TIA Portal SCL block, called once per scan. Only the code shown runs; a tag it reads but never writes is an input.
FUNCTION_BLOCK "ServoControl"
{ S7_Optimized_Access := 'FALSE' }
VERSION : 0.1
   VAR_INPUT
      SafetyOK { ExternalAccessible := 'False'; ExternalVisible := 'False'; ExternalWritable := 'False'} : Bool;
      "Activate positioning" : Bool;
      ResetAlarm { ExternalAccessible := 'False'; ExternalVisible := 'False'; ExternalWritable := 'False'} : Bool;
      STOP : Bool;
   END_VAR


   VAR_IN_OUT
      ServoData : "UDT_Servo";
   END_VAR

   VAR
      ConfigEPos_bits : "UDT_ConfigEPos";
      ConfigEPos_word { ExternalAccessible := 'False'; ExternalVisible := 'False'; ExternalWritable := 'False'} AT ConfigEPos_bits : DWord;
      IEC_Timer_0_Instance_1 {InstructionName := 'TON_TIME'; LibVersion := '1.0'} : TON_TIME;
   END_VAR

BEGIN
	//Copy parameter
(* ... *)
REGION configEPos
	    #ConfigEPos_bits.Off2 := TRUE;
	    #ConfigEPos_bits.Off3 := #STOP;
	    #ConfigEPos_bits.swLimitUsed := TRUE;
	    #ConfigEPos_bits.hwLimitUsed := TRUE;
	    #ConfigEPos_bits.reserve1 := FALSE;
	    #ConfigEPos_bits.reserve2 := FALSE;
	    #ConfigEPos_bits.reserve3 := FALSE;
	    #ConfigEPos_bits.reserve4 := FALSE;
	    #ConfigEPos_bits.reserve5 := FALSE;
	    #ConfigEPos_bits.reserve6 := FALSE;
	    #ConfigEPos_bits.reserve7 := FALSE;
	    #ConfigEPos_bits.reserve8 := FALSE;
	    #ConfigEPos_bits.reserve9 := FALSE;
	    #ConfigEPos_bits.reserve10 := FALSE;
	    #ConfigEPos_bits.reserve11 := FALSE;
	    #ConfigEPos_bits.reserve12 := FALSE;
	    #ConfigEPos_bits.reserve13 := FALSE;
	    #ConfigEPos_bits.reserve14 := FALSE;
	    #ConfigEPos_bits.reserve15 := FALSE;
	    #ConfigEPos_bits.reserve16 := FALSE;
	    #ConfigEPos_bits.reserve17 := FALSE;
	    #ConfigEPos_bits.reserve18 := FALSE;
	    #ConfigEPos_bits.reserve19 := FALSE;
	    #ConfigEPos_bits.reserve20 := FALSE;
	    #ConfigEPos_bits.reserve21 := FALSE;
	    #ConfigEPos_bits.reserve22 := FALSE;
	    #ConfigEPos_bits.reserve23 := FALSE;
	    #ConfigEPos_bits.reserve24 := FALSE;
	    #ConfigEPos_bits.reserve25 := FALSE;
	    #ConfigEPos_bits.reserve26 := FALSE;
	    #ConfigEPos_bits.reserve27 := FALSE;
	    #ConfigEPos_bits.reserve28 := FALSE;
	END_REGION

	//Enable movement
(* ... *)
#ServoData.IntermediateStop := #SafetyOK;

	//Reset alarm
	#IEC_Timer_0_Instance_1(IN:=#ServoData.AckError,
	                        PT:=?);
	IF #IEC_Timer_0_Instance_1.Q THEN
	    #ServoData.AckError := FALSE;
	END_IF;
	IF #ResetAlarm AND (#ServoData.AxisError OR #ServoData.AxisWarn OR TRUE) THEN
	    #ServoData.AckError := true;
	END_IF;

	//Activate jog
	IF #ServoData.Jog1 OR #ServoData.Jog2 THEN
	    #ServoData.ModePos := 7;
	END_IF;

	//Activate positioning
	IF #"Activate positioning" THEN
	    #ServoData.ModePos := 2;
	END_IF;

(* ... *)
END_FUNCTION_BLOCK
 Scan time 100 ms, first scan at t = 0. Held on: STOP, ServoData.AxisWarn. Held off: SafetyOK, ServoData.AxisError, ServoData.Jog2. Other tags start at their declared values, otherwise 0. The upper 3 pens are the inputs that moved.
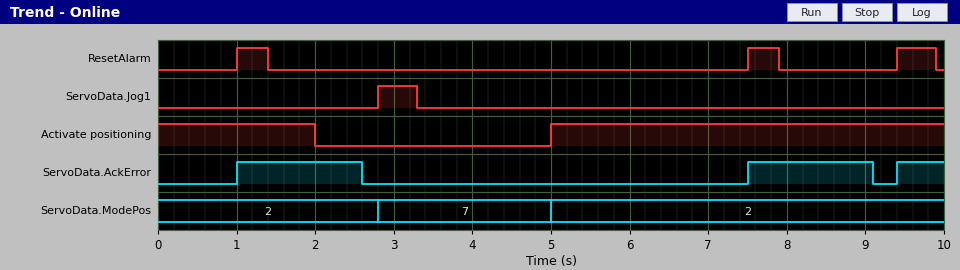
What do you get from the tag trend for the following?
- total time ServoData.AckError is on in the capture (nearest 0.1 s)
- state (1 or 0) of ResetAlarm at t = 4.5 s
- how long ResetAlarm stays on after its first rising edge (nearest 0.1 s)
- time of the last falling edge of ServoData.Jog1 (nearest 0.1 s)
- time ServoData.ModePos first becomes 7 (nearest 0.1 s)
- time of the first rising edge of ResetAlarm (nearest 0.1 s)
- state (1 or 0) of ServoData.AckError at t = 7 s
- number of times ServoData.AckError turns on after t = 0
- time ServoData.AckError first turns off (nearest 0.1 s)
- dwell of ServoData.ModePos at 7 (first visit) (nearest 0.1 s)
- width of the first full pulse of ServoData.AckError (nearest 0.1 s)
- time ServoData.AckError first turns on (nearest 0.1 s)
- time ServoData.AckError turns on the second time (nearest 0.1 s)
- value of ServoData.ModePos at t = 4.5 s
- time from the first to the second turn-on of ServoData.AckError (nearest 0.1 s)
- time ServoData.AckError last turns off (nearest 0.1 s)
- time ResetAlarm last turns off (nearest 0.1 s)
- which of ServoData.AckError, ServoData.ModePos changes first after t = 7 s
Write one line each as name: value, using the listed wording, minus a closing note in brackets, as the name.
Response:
total time ServoData.AckError is on in the capture: 3.8 s
state (1 or 0) of ResetAlarm at t = 4.5 s: 0
how long ResetAlarm stays on after its first rising edge: 0.4 s
time of the last falling edge of ServoData.Jog1: 3.3 s
time ServoData.ModePos first becomes 7: 2.8 s
time of the first rising edge of ResetAlarm: 1.0 s
state (1 or 0) of ServoData.AckError at t = 7 s: 0
number of times ServoData.AckError turns on after t = 0: 3
time ServoData.AckError first turns off: 2.6 s
dwell of ServoData.ModePos at 7 (first visit): 2.2 s
width of the first full pulse of ServoData.AckError: 1.6 s
time ServoData.AckError first turns on: 1.0 s
time ServoData.AckError turns on the second time: 7.5 s
value of ServoData.ModePos at t = 4.5 s: 7
time from the first to the second turn-on of ServoData.AckError: 6.5 s
time ServoData.AckError last turns off: 9.1 s
time ResetAlarm last turns off: 9.9 s
which of ServoData.AckError, ServoData.ModePos changes first after t = 7 s: ServoData.AckError
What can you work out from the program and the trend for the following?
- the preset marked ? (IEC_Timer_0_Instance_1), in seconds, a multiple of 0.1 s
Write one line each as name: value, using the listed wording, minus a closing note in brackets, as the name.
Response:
the preset marked ? (IEC_Timer_0_Instance_1), in seconds, a multiple of 0.1 s: 1.5 s
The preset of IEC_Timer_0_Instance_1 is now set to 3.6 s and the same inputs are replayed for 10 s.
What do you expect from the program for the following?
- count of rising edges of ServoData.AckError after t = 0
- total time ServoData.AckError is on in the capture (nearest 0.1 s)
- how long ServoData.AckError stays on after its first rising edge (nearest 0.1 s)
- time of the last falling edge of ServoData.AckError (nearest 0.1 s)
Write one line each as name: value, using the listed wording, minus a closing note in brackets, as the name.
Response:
count of rising edges of ServoData.AckError after t = 0: 2
total time ServoData.AckError is on in the capture: 6.2 s
how long ServoData.AckError stays on after its first rising edge: 3.7 s
time of the last falling edge of ServoData.AckError: 4.7 s
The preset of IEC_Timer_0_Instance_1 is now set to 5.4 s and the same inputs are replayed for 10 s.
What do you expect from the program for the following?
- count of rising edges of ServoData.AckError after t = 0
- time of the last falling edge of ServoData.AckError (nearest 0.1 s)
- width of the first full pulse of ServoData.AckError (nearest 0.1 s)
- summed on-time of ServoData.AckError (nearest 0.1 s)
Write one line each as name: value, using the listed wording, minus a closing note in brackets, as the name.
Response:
count of rising edges of ServoData.AckError after t = 0: 2
time of the last falling edge of ServoData.AckError: 6.5 s
width of the first full pulse of ServoData.AckError: 5.5 s
summed on-time of ServoData.AckError: 8.0 s
